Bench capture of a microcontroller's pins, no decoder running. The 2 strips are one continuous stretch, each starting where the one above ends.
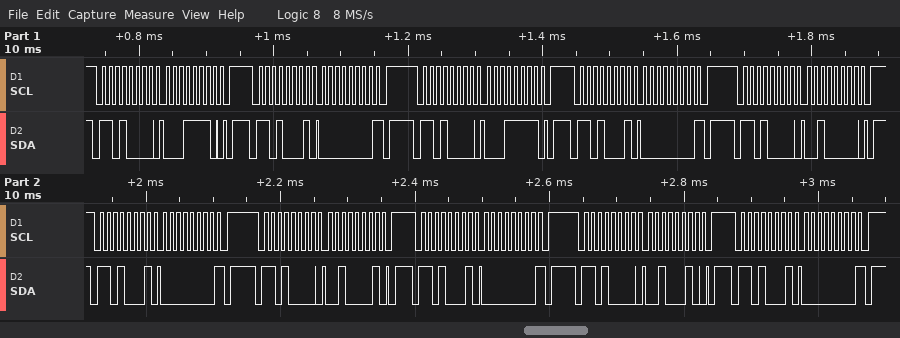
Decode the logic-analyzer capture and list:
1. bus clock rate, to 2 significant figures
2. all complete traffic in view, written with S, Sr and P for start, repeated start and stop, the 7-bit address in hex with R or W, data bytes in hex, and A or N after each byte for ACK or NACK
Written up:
100 kHz
S 68W A 1E A P S 68R A 00 N P S 68W A 1F A P S 68R A 00 N P S 68W A 20 A P S 68R A 00 N P S 68W A 21 A P S 68R A 00 N P S 68W A 22 A P S 68R A 00 N P
